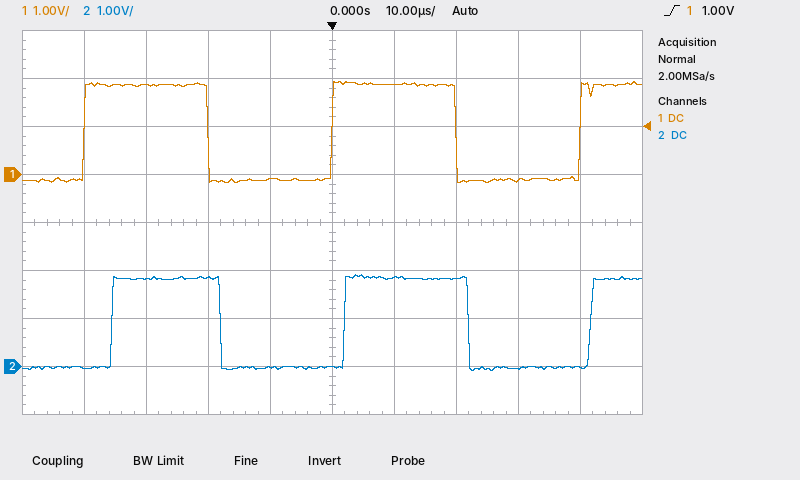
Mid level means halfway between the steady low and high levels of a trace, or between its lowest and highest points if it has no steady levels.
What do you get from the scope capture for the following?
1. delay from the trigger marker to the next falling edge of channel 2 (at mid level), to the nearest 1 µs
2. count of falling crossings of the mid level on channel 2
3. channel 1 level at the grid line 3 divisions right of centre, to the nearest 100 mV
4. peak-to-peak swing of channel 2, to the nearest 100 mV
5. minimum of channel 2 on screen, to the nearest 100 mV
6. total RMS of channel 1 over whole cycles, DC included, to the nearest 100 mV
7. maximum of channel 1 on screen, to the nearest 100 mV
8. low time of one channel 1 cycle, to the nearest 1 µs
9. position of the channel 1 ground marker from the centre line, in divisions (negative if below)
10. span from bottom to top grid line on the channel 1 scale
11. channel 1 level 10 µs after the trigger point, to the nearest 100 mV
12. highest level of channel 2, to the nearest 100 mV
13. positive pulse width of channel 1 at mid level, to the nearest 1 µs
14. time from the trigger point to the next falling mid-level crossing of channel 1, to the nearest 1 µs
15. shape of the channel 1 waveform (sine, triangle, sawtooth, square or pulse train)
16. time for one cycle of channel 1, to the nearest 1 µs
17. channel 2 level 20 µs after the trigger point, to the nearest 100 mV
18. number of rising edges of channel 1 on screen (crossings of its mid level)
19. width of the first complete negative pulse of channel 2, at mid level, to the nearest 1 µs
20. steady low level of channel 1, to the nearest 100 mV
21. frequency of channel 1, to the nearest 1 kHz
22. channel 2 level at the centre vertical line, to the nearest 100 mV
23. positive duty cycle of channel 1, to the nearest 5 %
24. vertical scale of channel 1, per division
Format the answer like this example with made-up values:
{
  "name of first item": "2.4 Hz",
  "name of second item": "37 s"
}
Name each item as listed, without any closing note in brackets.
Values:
{
  "delay from the trigger marker to the next falling edge of channel 2 (at mid level), to the nearest 1 µs": "22 µs",
  "count of falling crossings of the mid level on channel 2": "2",
  "channel 1 level at the grid line 3 divisions right of centre, to the nearest 100 mV": "-100 mV",
  "peak-to-peak swing of channel 2, to the nearest 100 mV": "2.0 V",
  "minimum of channel 2 on screen, to the nearest 100 mV": "-100 mV",
  "total RMS of channel 1 over whole cycles, DC included, to the nearest 100 mV": "1.3 V",
  "maximum of channel 1 on screen, to the nearest 100 mV": "1.9 V",
  "low time of one channel 1 cycle, to the nearest 1 µs": "20 µs",
  "position of the channel 1 ground marker from the centre line, in divisions": "+1.0 div",
  "span from bottom to top grid line on the channel 1 scale": "8 V",
  "channel 1 level 10 µs after the trigger point, to the nearest 100 mV": "1.9 V",
  "highest level of channel 2, to the nearest 100 mV": "1.9 V",
  "positive pulse width of channel 1 at mid level, to the nearest 1 µs": "20 µs",
  "time from the trigger point to the next falling mid-level crossing of channel 1, to the nearest 1 µs": "20 µs",
  "shape of the channel 1 waveform": "square",
  "time for one cycle of channel 1, to the nearest 1 µs": "40 µs",
  "channel 2 level 20 µs after the trigger point, to the nearest 100 mV": "1.8 V",
  "number of rising edges of channel 1 on screen": "3",
  "width of the first complete negative pulse of channel 2, at mid level, to the nearest 1 µs": "20 µs",
  "steady low level of channel 1, to the nearest 100 mV": "-100 mV",
  "frequency of channel 1, to the nearest 1 kHz": "25 kHz",
  "channel 2 level at the centre vertical line, to the nearest 100 mV": "0.0 V",
  "positive duty cycle of channel 1, to the nearest 5 %": "50 %",
  "vertical scale of channel 1, per division": "1 V"
}
